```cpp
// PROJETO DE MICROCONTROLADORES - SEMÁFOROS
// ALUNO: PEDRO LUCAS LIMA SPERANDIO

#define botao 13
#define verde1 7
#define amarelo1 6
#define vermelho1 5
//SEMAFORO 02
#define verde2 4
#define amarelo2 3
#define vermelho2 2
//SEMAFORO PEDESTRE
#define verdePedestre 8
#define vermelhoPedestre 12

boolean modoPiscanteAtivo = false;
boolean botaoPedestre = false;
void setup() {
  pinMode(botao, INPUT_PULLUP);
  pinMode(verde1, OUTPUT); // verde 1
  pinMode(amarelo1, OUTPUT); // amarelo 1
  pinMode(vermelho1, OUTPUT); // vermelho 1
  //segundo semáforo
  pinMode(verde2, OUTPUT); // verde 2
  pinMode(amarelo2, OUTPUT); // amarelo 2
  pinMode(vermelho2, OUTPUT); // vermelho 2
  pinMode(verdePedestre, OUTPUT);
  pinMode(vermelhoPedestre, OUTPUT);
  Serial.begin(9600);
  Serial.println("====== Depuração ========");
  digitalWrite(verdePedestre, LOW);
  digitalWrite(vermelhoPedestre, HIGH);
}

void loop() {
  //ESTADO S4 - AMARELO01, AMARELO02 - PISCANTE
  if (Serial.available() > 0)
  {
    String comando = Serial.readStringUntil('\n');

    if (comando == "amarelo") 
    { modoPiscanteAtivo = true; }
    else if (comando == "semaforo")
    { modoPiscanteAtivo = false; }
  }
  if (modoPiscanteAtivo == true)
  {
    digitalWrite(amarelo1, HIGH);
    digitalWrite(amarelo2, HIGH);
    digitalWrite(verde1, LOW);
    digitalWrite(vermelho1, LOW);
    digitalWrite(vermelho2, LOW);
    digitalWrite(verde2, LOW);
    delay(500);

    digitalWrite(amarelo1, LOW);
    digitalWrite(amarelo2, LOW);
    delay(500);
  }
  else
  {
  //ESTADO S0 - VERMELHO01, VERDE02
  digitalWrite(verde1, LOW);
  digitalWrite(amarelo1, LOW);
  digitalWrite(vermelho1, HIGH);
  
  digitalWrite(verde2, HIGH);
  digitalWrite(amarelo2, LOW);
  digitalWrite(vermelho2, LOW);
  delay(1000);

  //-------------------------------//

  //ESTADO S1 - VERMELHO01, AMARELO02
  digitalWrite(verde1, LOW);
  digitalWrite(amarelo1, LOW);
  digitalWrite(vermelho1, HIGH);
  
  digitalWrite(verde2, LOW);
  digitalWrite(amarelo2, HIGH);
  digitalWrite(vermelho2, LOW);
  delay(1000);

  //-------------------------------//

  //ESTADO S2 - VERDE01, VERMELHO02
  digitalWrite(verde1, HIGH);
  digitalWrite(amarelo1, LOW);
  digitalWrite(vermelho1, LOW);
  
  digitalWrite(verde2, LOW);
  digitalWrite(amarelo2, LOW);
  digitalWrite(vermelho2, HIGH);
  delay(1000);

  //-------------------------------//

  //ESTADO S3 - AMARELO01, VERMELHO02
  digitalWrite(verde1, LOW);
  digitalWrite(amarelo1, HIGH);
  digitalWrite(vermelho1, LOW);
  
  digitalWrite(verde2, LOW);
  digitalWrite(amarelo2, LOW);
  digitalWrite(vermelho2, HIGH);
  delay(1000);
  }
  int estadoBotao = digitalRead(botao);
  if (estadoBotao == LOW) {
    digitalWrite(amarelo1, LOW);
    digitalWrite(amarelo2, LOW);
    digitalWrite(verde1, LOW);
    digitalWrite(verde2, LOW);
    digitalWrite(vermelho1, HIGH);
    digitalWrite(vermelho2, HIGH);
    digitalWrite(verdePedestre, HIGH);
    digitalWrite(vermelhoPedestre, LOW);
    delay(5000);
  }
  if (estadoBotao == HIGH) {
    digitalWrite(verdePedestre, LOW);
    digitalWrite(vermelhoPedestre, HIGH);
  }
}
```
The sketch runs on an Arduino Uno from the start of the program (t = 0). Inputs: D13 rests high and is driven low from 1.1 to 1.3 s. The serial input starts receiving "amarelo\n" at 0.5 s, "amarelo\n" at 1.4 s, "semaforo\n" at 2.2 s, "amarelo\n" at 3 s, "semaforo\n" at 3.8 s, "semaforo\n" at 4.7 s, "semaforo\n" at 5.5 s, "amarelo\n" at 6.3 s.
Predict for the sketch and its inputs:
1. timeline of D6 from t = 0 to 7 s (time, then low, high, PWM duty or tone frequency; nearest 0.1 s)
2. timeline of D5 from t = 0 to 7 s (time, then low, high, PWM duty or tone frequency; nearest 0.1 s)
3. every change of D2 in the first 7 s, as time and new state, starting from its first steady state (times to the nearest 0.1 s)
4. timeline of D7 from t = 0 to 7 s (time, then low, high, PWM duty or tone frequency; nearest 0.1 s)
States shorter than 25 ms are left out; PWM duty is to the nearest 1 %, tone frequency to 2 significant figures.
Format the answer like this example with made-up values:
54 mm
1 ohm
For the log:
0 s low; 3 s high; 4.5 s low; 5 s high; 5.5 s low
0 s high; 2 s low; 6 s high
0 s low; 2 s high; 4 s low
0 s low; 2 s high; 3 s low
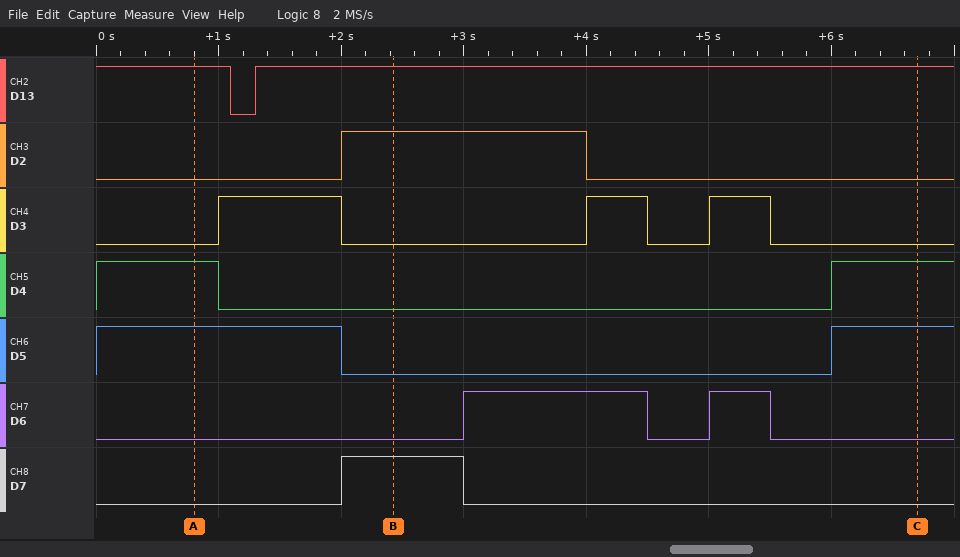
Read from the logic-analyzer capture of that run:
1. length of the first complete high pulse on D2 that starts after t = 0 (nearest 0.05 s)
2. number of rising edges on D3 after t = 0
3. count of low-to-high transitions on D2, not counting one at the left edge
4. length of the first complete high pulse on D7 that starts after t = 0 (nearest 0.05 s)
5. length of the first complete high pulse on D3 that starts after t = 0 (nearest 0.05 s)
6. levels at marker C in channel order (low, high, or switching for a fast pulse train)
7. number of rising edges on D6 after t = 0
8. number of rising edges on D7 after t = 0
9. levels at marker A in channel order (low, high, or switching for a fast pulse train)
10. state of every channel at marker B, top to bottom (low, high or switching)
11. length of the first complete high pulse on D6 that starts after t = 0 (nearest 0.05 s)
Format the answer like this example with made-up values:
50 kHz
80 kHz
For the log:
2.00 s
3
1
1.00 s
1.00 s
D13 high, D2 low, D3 low, D4 high, D5 high, D6 low, D7 low
2
1
D13 high, D2 low, D3 low, D4 high, D5 high, D6 low, D7 low
D13 high, D2 high, D3 low, D4 low, D5 low, D6 low, D7 high
1.50 s
